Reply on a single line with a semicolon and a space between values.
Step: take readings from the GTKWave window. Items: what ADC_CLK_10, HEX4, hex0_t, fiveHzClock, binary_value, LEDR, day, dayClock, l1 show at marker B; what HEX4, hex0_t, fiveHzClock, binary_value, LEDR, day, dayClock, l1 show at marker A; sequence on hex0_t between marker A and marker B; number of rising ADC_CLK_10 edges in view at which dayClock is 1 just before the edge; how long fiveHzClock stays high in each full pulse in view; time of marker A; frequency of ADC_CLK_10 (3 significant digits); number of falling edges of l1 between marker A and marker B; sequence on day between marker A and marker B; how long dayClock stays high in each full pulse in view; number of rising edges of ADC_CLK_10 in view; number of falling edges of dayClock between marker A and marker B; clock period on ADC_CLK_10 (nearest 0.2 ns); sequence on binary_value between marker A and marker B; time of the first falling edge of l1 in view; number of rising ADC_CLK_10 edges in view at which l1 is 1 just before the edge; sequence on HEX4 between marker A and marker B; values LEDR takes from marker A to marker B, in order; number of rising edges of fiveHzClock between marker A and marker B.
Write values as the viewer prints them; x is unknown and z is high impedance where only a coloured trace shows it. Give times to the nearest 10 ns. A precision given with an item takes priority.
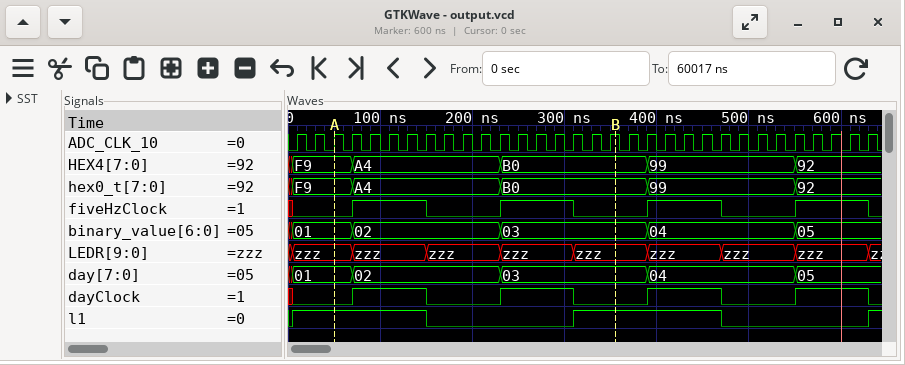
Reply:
ADC_CLK_10=1, HEX4=B0, hex0_t=B0, fiveHzClock=0, binary_value=03, LEDR=zzz, day=03, dayClock=0, l1=1; HEX4=F9, hex0_t=F9, fiveHzClock=0, binary_value=01, LEDR=zzz, day=01, dayClock=0, l1=1; F9, A4, B0; 16; 80 ns, 80 ns, 80 ns, 80 ns; 50 ns; 50.0 MHz; 1; 01, 02, 03; 80 ns, 80 ns, 80 ns, 80 ns; 32; 2; 20 ns; 01, 02, 03; 150 ns; 16; F9, A4, B0; zzz, zzz, zzz, zzz, zzz; 2
